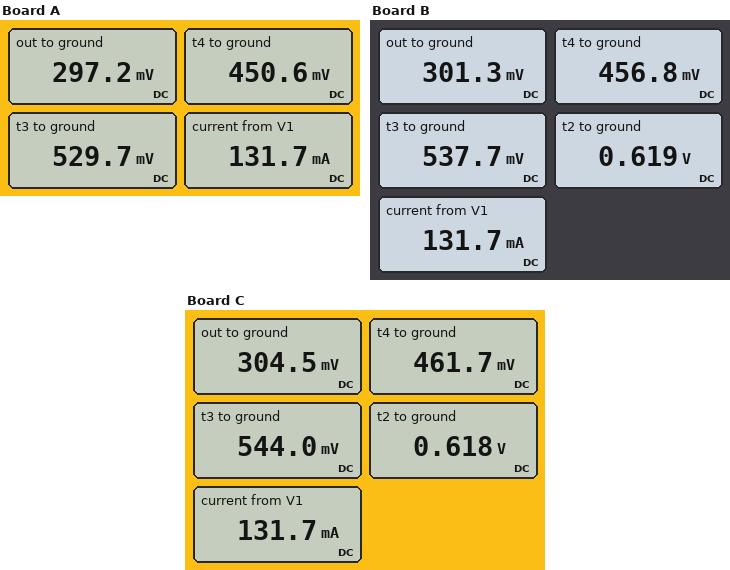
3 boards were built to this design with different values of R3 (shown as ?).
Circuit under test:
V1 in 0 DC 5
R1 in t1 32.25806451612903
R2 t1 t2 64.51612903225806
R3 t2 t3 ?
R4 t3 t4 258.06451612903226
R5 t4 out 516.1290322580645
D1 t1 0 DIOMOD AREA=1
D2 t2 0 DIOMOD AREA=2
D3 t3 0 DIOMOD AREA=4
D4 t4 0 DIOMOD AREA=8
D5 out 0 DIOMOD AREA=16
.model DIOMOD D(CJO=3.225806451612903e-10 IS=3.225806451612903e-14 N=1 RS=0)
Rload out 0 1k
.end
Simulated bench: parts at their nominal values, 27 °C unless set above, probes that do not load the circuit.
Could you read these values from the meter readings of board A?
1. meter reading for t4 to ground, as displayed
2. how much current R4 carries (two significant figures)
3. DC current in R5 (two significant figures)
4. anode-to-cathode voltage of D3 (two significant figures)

450.6 mV
310 µA
300 µA
530 mV
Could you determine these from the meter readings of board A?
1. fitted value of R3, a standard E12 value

220 Ω
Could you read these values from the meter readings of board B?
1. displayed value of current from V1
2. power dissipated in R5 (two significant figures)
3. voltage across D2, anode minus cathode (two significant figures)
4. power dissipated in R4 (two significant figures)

131.7 mA
47 µW
620 mV
25 µW
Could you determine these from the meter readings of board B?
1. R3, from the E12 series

180 Ω
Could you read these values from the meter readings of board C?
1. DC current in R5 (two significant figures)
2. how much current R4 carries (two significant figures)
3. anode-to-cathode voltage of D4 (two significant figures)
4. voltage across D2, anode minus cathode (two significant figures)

300 µA
320 µA
460 mV
620 mV
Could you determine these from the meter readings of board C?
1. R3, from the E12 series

150 Ω
